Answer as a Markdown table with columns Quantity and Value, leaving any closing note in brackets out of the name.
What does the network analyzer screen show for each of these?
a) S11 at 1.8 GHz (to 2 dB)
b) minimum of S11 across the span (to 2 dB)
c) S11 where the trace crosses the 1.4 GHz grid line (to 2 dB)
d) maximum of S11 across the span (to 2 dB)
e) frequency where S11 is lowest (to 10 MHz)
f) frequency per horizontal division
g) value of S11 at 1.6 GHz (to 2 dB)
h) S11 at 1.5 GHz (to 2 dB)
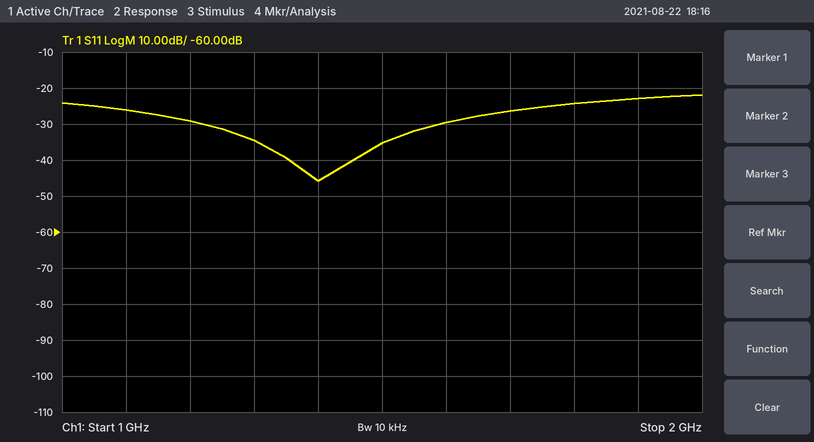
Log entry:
| Quantity | Value |
|---|---|
| S11 at 1.8 GHz | -24 dB |
| minimum of S11 across the span | -46 dB |
| S11 where the trace crosses the 1.4 GHz grid line | -46 dB |
| maximum of S11 across the span | -22 dB |
| frequency where S11 is lowest | 1.40 GHz |
| frequency per horizontal division | 100 MHz |
| value of S11 at 1.6 GHz | -30 dB |
| S11 at 1.5 GHz | -36 dB |
